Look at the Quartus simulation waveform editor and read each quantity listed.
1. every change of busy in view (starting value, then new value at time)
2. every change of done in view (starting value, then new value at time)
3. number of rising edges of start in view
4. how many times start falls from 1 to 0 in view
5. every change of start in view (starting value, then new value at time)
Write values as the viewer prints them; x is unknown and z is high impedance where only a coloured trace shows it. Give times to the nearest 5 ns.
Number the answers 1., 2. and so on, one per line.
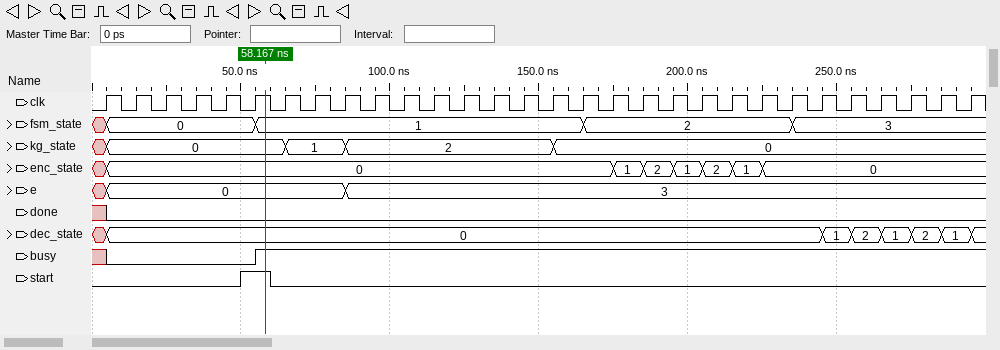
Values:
1. x, 0 at 5 ns, 1 at 55 ns
2. x, 0 at 5 ns
3. 1
4. 1
5. 0, 1 at 50 ns, 0 at 60 ns
